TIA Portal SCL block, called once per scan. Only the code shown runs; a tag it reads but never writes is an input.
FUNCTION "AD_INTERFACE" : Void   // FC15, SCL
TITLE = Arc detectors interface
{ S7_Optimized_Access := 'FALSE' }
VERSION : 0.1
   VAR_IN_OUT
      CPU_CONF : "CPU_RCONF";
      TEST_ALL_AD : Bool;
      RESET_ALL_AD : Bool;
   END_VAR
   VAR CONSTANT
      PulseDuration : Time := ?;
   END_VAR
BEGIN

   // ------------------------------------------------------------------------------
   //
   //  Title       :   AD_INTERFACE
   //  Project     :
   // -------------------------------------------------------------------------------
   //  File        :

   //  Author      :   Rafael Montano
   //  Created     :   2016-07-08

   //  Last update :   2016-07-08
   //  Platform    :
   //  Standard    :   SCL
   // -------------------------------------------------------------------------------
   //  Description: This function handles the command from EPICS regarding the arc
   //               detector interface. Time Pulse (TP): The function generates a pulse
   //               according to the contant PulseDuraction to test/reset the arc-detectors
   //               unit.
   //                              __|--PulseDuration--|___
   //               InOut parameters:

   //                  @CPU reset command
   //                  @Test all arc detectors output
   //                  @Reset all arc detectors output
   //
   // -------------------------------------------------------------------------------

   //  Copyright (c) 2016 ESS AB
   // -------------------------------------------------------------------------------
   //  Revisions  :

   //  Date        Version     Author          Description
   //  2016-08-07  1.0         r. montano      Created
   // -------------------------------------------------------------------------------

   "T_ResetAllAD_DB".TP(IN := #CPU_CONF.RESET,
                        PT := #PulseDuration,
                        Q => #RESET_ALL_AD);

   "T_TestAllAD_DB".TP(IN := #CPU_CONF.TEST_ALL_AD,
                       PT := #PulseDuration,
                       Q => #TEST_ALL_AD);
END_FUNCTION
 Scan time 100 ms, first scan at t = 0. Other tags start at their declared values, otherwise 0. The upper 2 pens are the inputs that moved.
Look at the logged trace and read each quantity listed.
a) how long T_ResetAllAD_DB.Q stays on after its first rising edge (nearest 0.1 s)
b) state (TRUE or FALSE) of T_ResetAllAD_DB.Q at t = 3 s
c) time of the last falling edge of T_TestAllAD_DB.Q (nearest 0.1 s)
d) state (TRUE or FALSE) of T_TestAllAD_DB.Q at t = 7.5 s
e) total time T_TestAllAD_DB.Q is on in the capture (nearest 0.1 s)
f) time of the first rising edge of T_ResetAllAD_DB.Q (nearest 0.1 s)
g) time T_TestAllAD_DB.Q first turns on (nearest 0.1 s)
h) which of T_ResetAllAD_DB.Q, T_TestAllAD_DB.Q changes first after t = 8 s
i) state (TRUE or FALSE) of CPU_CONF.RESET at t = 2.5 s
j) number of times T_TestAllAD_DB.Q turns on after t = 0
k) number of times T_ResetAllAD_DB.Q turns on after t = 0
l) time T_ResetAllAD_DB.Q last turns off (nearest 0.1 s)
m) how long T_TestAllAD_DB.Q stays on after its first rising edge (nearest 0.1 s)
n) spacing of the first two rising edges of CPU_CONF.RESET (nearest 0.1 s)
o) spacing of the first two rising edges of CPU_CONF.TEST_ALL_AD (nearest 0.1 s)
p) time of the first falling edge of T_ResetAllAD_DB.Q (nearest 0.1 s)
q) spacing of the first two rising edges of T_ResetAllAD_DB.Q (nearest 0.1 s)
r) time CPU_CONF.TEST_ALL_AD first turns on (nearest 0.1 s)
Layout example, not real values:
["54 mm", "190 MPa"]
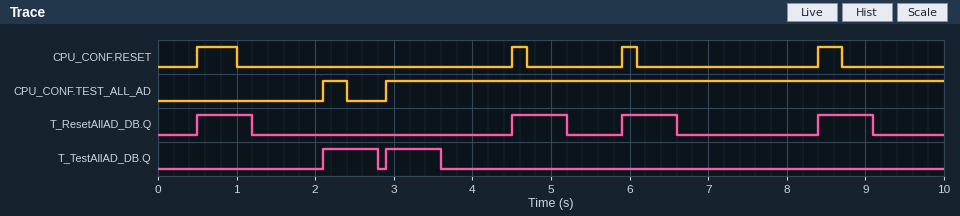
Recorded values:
["0.7 s", "FALSE", "3.6 s", "FALSE", "1.4 s", "0.5 s", "2.1 s", "T_ResetAllAD_DB.Q", "FALSE", "2", "4", "9.1 s", "0.7 s", "4.0 s", "0.8 s", "1.2 s", "4.0 s", "2.1 s"]
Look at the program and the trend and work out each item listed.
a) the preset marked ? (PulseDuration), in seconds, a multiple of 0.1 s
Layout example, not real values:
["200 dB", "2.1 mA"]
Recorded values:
["0.7 s"]
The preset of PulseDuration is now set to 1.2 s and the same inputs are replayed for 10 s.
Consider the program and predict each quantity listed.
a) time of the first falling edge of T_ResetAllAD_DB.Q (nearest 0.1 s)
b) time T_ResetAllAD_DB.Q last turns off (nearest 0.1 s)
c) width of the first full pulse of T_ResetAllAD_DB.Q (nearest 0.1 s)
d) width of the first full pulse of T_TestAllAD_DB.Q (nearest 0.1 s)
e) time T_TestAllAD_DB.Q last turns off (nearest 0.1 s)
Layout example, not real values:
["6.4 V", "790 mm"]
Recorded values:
["1.7 s", "9.6 s", "1.2 s", "1.2 s", "3.3 s"]
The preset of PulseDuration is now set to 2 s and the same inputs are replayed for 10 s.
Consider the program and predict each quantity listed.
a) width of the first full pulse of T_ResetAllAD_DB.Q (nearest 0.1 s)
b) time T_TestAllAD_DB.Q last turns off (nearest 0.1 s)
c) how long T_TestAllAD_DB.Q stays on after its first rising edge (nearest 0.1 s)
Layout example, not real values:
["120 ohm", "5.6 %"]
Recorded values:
["2.0 s", "4.1 s", "2.0 s"]
